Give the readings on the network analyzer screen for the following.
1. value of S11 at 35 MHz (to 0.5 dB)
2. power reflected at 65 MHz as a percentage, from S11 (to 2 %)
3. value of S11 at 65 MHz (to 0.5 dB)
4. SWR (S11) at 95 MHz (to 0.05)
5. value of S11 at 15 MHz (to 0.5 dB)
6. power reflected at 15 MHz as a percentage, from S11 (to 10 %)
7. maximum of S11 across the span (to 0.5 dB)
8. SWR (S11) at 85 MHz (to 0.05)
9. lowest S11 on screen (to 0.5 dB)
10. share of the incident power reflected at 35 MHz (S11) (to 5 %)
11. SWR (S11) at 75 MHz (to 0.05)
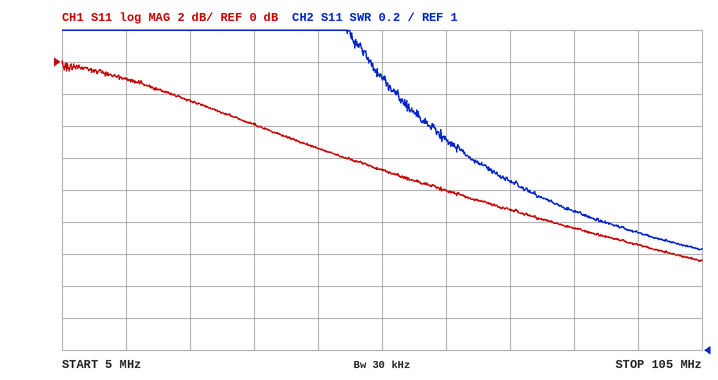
-4.0 dB
16 %
-8.0 dB
1.75
-1.0 dB
80 %
0.0 dB
1.85
-12.5 dB
40 %
2.05
